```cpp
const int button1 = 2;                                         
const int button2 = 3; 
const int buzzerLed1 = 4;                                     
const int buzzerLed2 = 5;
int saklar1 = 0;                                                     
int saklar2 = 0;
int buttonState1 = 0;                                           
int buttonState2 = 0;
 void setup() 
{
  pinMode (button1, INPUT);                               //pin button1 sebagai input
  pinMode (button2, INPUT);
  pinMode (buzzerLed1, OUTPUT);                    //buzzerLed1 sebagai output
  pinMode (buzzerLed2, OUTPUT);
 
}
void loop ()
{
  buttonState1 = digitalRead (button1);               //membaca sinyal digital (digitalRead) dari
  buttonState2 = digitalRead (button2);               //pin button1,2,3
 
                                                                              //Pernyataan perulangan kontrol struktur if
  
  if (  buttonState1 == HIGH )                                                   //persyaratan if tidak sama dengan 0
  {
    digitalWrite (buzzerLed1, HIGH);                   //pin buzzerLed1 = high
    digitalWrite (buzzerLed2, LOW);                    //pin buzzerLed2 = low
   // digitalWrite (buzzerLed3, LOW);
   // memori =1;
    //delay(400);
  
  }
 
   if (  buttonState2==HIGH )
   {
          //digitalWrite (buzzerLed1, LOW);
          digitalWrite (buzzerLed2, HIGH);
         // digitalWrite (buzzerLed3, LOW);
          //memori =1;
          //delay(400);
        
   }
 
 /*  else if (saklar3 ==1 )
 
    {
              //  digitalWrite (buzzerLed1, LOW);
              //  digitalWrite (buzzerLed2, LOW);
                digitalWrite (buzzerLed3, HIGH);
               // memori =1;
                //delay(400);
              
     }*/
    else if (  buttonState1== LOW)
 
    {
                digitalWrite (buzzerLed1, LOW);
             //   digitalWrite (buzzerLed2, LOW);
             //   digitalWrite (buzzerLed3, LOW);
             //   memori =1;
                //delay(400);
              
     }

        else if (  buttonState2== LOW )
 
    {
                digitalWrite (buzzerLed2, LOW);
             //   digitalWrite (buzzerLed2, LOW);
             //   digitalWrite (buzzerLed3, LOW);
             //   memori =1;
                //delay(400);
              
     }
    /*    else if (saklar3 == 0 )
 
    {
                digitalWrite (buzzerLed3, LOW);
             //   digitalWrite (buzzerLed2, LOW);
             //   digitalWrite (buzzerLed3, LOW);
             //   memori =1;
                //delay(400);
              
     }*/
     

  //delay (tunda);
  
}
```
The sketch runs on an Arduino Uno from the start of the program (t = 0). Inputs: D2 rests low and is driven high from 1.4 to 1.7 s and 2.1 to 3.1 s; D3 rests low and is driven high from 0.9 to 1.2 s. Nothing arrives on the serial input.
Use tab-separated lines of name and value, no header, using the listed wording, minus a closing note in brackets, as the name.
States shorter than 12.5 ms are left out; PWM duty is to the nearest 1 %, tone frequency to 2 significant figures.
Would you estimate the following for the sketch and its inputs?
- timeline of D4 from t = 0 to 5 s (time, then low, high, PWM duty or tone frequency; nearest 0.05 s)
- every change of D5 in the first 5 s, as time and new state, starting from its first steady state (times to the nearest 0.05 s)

timeline of D4 from t = 0 to 5 s	0 s low; 1.4 s high; 1.7 s low; 2.1 s high; 3.1 s low
every change of D5 in the first 5 s, as time and new state, starting from its first steady state	0 s low; 0.9 s high; 1.4 s low
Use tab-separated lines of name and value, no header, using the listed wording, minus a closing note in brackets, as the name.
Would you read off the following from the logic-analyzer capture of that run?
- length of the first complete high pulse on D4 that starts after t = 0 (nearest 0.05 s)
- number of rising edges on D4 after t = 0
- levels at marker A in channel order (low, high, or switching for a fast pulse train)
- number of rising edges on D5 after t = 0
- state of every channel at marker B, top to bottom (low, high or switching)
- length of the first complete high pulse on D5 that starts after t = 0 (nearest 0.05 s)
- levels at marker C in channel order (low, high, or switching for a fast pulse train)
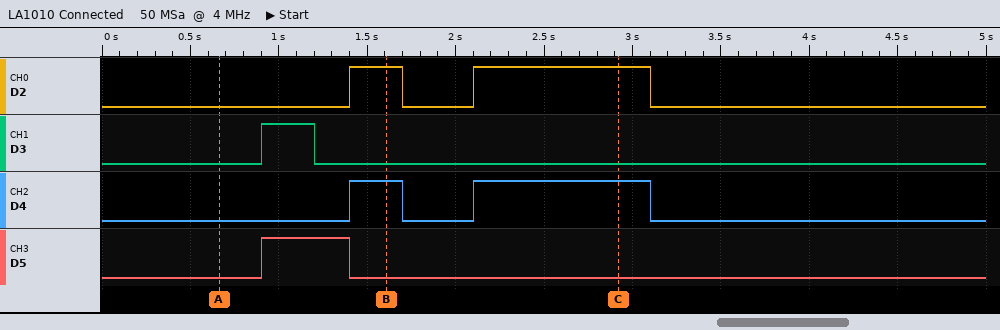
length of the first complete high pulse on D4 that starts after t = 0	0.30 s
number of rising edges on D4 after t = 0	2
levels at marker A in channel order	D2 low, D3 low, D4 low, D5 low
number of rising edges on D5 after t = 0	1
state of every channel at marker B, top to bottom	D2 high, D3 low, D4 high, D5 low
length of the first complete high pulse on D5 that starts after t = 0	0.50 s
levels at marker C in channel order	D2 high, D3 low, D4 high, D5 low
